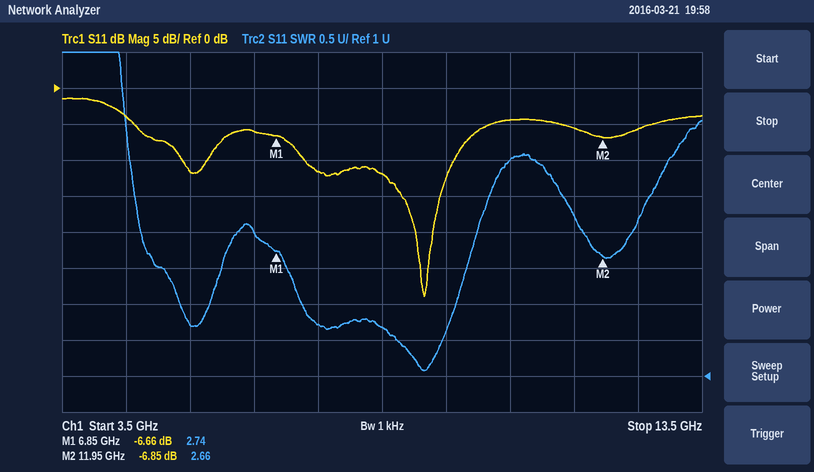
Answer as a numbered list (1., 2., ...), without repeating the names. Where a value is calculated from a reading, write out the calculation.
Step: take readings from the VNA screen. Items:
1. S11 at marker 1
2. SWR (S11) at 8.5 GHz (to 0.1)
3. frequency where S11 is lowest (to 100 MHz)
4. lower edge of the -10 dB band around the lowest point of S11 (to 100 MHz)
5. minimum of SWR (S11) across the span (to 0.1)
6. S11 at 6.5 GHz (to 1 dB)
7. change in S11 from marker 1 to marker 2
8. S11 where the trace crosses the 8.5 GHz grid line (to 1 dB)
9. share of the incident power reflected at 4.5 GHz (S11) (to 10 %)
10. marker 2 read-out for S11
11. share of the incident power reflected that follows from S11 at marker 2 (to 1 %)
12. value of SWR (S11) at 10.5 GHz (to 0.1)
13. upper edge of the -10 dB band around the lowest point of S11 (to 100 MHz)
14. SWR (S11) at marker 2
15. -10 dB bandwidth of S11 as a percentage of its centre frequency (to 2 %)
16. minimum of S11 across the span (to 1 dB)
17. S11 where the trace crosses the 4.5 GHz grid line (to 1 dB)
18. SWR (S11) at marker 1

1. -6.66 dB
2. 1.7
3. 9.2 GHz
4. 7.3 GHz
5. 1.1
6. -6 dB
7. -6.85 − (-6.66) = -0.19 dB
8. -12 dB
9. 10^(-4/10) ≈ 40 %
10. -6.85 dB
11. 10^(-6.85/10) ≈ 21 %
12. 4.0
13. 9.6 GHz
14. 2.66
15. 2.3 GHz / 8.45 GHz ≈ 27.2 %, so 28 % to the nearest 2 %
16. -29 dB
17. -4 dB
18. 2.74
